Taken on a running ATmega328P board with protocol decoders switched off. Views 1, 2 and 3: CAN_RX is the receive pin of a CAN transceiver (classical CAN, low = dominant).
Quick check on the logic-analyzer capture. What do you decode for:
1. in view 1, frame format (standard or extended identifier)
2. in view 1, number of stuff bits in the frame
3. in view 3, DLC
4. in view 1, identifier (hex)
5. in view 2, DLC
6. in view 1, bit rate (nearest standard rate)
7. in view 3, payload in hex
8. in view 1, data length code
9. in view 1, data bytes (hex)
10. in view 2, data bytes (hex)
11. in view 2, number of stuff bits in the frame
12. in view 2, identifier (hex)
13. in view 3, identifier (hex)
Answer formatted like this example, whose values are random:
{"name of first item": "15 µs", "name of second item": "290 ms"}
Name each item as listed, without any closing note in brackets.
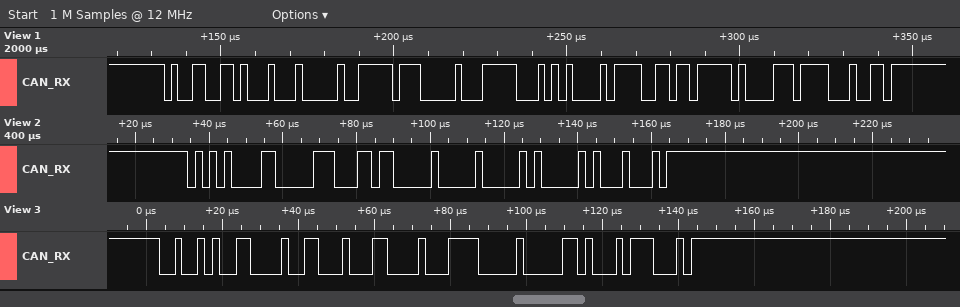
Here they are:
{"in view 1, frame format": "standard", "in view 1, number of stuff bits in the frame": "5", "in view 3, DLC": "4", "in view 1, identifier": "0x4CD", "in view 2, DLC": "3", "in view 1, bit rate": "500 kbit/s", "in view 3, payload in hex": "C4 61 1E 00", "in view 1, data length code": "8", "in view 1, data bytes": "80 FF 00 F9 50 BC DB F0", "in view 2, data bytes": "1B 00 00", "in view 2, number of stuff bits in the frame": "5", "in view 2, identifier": "0x543", "in view 3, identifier": "0x253"}
